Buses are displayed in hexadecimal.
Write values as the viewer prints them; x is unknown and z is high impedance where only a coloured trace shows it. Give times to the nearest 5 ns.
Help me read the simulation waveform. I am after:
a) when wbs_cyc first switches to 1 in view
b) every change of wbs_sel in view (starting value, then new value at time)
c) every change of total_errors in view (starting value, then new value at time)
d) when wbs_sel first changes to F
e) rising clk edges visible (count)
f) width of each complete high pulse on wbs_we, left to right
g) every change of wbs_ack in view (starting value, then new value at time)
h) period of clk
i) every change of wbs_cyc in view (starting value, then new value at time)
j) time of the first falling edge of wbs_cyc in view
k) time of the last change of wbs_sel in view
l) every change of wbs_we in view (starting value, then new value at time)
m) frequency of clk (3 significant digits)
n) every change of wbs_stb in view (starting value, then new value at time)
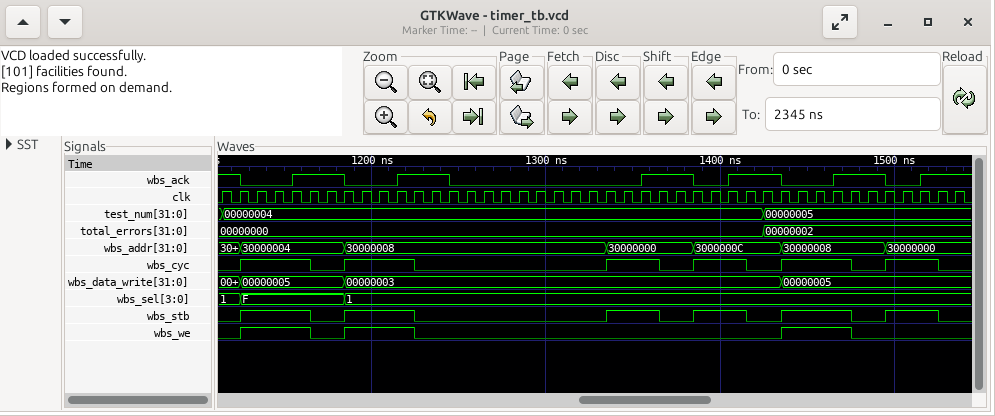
1125 ns
1, F at 1125 ns, 1 at 1185 ns
00000000, 00000002 at 1425 ns
1125 ns
43
40 ns, 40 ns, 40 ns
1, 0 at 1125 ns, 1 at 1155 ns, 0 at 1185 ns, 1 at 1215 ns, 0 at 1245 ns, 1 at 1355 ns, 0 at 1385 ns, 1 at 1405 ns, 0 at 1435 ns, 1 at 1465 ns, 0 at 1495 ns, 1 at 1515 ns
10 ns
0, 1 at 1125 ns, 0 at 1165 ns, 1 at 1185 ns, 0 at 1225 ns, 1 at 1335 ns, 0 at 1365 ns, 1 at 1385 ns, 0 at 1415 ns, 1 at 1435 ns, 0 at 1475 ns, 1 at 1495 ns, 0 at 1525 ns
1165 ns
1185 ns
0, 1 at 1125 ns, 0 at 1165 ns, 1 at 1185 ns, 0 at 1225 ns, 1 at 1435 ns, 0 at 1475 ns
100 MHz
0, 1 at 1125 ns, 0 at 1165 ns, 1 at 1185 ns, 0 at 1225 ns, 1 at 1335 ns, 0 at 1365 ns, 1 at 1385 ns, 0 at 1415 ns, 1 at 1435 ns, 0 at 1475 ns, 1 at 1495 ns, 0 at 1525 ns
